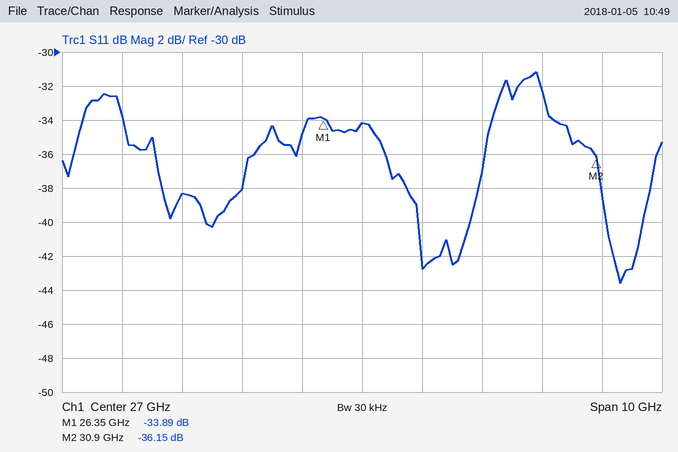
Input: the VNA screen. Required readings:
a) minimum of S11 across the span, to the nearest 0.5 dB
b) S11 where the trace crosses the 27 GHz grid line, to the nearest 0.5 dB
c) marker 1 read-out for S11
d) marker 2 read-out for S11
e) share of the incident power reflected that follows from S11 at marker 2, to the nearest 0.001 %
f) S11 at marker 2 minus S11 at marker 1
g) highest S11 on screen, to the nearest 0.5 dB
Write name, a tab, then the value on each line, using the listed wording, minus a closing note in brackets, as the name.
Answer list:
minimum of S11 across the span, to the nearest 0.5 dB	-43.5 dB
S11 where the trace crosses the 27 GHz grid line, to the nearest 0.5 dB	-34.0 dB
marker 1 read-out for S11	-33.89 dB
marker 2 read-out for S11	-36.15 dB
share of the incident power reflected that follows from S11 at marker 2, to the nearest 0.001 %	0.024 %
S11 at marker 2 minus S11 at marker 1	-2.26 dB
highest S11 on screen, to the nearest 0.5 dB	-31.0 dB
